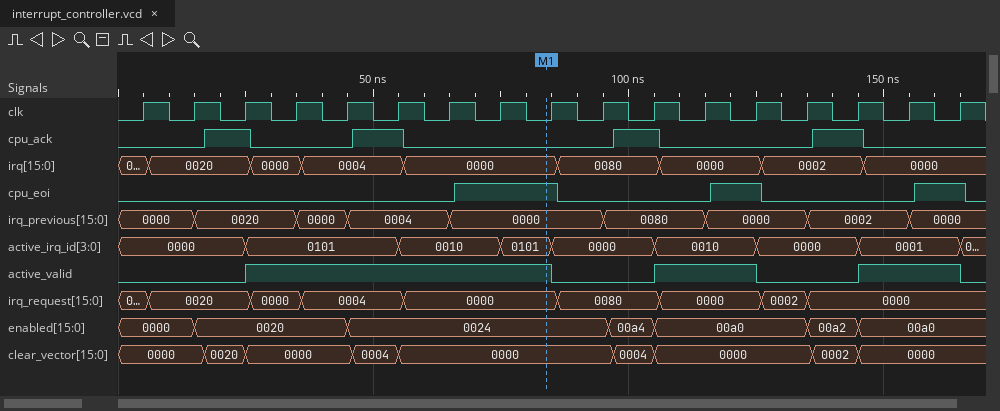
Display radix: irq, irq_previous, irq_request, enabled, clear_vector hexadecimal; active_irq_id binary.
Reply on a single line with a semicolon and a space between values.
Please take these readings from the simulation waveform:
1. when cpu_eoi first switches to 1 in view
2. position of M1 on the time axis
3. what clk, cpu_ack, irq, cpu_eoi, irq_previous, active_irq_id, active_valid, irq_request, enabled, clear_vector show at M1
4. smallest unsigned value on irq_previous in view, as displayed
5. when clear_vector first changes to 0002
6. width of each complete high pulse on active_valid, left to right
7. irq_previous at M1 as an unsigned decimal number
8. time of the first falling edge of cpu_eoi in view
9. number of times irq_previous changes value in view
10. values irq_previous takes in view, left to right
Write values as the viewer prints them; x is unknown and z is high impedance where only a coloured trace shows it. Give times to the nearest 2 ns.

66 ns; 84 ns; clk=0, cpu_ack=0, irq=0000, cpu_eoi=1, irq_previous=0000, active_irq_id=0101, active_valid=1, irq_request=0000, enabled=0024, clear_vector=0000; 0000; 136 ns; 60 ns, 20 ns, 20 ns; 0; 86 ns; 8; 0000, 0020, 0000, 0004, 0000, 0080, 0000, 0002, 0000
